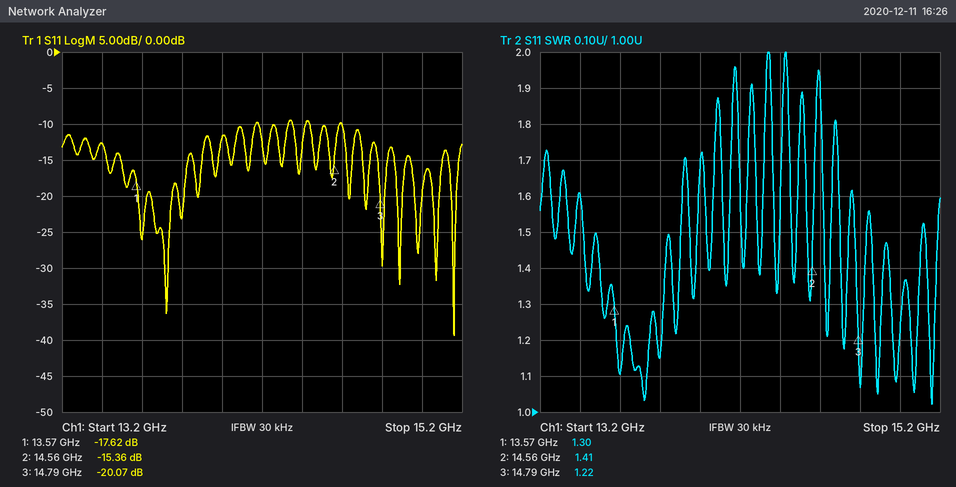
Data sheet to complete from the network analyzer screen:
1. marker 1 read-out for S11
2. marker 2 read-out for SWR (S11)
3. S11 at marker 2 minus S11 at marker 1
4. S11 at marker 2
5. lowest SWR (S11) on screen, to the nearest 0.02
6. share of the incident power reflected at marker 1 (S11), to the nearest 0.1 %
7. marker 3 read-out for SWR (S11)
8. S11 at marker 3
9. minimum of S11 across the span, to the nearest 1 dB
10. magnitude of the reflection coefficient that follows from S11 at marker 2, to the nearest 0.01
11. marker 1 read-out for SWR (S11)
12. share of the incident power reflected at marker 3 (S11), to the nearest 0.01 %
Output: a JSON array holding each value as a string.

["-17.62 dB", "1.41", "2.26 dB", "-15.36 dB", "1.02", "1.7 %", "1.22", "-20.07 dB", "-39 dB", "0.17", "1.30", "0.98 %"]
